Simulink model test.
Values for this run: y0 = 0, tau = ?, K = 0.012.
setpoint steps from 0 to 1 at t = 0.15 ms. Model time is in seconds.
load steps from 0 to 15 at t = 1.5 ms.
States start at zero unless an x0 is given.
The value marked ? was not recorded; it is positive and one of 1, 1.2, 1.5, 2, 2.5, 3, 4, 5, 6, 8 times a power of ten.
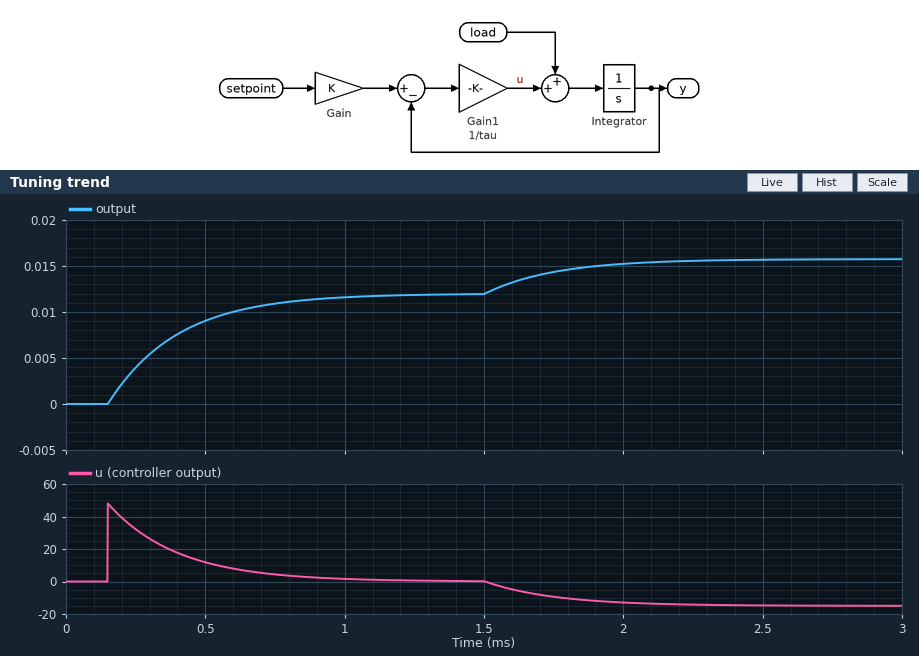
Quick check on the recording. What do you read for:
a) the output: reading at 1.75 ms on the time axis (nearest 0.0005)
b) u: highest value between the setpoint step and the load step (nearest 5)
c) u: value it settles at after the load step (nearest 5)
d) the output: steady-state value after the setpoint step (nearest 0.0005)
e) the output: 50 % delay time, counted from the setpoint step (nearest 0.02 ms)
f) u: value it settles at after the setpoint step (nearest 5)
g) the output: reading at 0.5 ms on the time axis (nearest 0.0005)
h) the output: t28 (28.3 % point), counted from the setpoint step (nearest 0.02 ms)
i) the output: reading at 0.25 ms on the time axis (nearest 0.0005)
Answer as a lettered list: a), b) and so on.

a) 0.0145
b) 50
c) -15
d) 0.0120
e) 0.18 ms
f) 0
g) 0.0090
h) 0.08 ms
i) 0.0040
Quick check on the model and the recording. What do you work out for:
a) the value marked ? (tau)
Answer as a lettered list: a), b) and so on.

a) 0.00025
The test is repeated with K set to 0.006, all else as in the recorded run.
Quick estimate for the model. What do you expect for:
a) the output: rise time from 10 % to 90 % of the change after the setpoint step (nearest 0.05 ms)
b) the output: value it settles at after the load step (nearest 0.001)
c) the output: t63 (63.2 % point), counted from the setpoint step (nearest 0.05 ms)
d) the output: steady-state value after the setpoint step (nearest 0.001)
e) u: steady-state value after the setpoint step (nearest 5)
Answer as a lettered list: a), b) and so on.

a) 0.55 ms
b) 0.010
c) 0.25 ms
d) 0.006
e) 0
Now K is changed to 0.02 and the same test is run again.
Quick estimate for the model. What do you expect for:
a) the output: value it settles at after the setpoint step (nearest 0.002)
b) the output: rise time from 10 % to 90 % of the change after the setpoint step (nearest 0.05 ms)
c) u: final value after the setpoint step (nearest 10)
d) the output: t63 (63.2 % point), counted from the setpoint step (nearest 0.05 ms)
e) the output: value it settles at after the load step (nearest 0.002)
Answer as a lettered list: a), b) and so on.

a) 0.020
b) 0.55 ms
c) 0
d) 0.25 ms
e) 0.024
